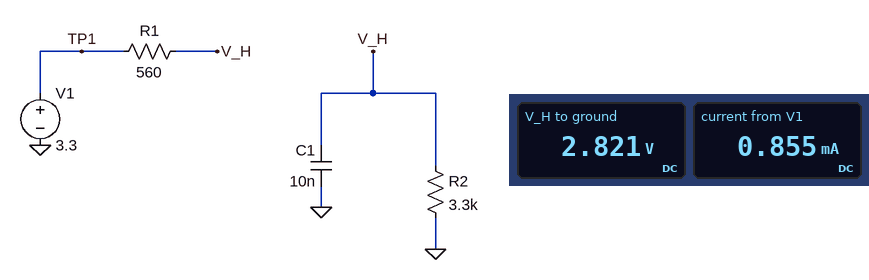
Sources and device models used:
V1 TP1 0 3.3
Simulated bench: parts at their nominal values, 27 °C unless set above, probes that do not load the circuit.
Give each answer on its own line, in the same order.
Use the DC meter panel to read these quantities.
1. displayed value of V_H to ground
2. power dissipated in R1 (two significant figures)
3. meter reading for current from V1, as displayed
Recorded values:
2.821 V
410 µW
0.855 mA
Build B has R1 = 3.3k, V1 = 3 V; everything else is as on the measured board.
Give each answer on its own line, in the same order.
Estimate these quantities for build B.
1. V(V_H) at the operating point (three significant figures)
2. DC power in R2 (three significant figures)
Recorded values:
1.50 V
682 µW
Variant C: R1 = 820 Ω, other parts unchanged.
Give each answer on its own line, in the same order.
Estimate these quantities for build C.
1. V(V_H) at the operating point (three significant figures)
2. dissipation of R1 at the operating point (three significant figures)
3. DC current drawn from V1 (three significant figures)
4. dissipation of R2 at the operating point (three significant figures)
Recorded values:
2.64 V
526 µW
801 µA
2.12 mW
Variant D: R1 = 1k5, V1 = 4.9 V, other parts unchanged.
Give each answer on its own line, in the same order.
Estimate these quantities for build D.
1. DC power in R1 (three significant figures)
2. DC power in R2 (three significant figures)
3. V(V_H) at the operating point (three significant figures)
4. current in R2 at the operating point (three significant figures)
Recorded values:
1.56 mW
3.44 mW
3.37 V
1.02 mA
